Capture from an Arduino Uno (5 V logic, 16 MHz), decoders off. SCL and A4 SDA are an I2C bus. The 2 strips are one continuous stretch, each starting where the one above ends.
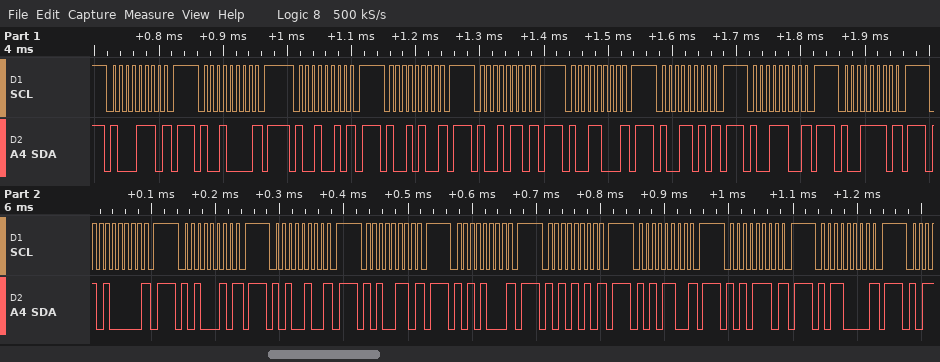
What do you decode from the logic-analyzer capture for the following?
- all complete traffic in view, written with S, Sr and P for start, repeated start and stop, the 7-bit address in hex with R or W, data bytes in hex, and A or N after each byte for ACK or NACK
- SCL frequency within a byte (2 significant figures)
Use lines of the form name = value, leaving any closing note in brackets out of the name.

all complete traffic in view, written with S, Sr and P for start, repeated start and stop, the 7-bit address in hex with R or W, data bytes in hex, and A or N after each byte for ACK or NACK = S 47W N P S 48W N P S 49W N P S 4AW N P S 4BW N P S 4CW N P S 4DW N P S 4EW N P S 4FW N P S 50W N P S 51W N P S 52W N P S 53W N P S 54W N P S 55W N P S 56W N P S 57W N P S 58W N P
SCL frequency within a byte = 100 kHz
